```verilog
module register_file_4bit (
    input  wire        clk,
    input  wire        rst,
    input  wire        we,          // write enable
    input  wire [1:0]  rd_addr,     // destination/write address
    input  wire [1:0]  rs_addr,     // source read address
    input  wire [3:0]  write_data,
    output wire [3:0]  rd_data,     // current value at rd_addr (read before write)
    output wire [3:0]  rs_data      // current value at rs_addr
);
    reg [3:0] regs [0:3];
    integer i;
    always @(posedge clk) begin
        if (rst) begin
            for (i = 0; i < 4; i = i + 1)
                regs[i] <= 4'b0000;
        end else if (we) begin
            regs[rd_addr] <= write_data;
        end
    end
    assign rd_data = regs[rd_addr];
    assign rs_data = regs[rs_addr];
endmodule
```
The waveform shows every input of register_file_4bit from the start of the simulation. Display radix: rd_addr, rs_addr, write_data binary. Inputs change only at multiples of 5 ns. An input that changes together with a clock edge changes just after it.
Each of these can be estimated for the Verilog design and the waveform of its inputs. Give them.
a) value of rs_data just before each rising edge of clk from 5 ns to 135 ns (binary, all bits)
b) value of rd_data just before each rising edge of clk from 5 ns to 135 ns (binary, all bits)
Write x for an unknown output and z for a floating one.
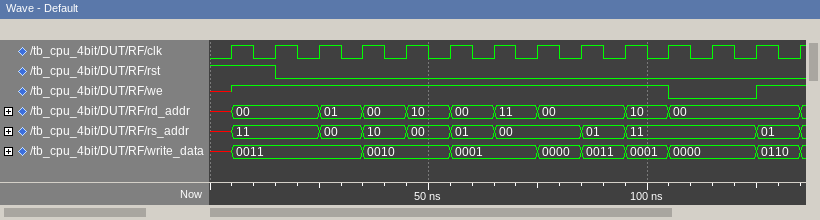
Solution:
x, 0000, 0000, 0011, 0000, 0010, 0011, 0001, 0001, 0011, 0001, 0001, 0001, 0011
x, 0000, 0000, 0000, 0011, 0000, 0010, 0000, 0001, 0000, 0010, 0011, 0011, 0011
